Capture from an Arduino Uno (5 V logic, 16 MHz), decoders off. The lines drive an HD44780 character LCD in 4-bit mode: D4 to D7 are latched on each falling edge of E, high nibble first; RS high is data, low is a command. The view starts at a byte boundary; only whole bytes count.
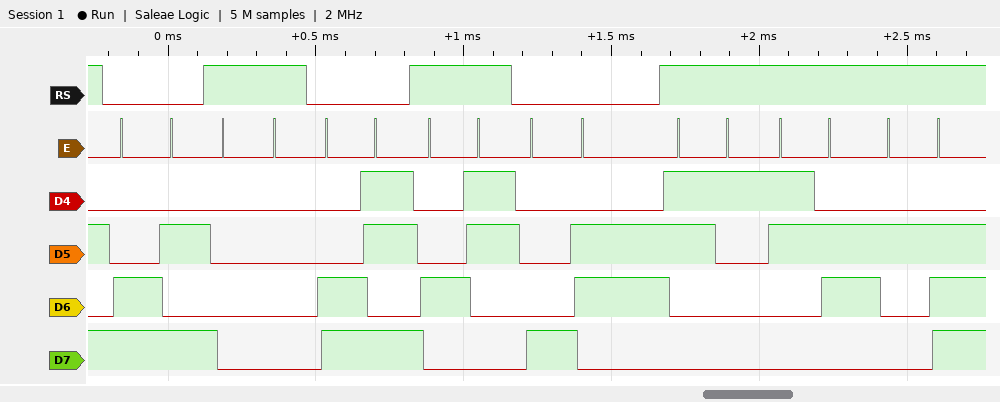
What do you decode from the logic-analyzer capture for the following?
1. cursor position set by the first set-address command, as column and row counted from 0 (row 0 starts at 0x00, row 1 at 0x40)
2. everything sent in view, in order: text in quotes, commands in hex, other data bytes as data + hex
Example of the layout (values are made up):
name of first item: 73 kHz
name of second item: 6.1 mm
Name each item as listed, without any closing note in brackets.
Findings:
cursor position set by the first set-address command, as column and row counted from 0: column 10, row 1
everything sent in view, in order: text in quotes, commands in hex, other data bytes as data + hex: 0xCA data 00 0xCB "C" 0x86 "16."
